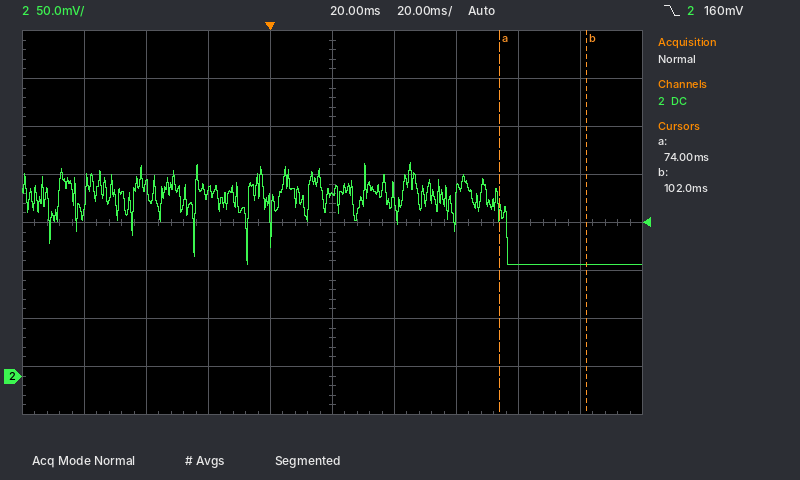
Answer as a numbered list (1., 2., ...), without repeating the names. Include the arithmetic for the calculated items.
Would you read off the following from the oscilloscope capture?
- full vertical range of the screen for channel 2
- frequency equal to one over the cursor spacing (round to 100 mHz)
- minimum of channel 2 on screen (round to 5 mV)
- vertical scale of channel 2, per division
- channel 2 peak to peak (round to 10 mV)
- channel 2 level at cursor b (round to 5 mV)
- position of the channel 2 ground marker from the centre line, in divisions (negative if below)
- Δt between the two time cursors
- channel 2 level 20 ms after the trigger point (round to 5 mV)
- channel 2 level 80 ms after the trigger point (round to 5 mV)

1. 400 mV
2. 1 / 28 ms ≈ 35.7 Hz
3. 115 mV
4. 50 mV
5. 110 mV
6. 115 mV
7. -3.2 div
8. 102 ms − (74 ms) = 28 ms
9. 190 mV
10. 115 mV
